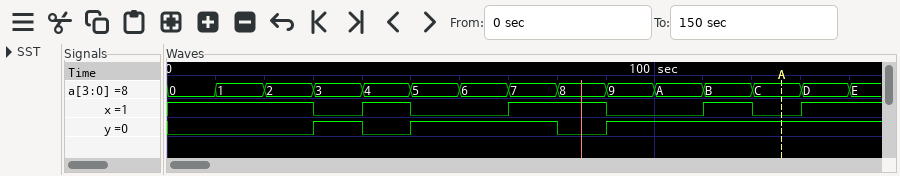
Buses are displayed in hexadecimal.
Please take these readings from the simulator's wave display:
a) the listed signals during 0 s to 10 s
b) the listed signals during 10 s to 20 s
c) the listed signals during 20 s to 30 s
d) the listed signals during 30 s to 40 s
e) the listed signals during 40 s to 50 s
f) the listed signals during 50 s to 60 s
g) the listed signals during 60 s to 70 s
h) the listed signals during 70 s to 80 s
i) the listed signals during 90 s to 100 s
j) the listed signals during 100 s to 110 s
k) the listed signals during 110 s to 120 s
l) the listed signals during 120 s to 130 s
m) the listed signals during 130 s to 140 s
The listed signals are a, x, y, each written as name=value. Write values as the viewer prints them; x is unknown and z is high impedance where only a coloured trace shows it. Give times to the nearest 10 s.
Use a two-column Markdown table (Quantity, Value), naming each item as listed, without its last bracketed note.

| Quantity | Value |
|---|---|
| the listed signals during 0 s to 10 s | a=0, x=1, y=0 |
| the listed signals during 10 s to 20 s | a=1, x=1, y=0 |
| the listed signals during 20 s to 30 s | a=2, x=1, y=0 |
| the listed signals during 30 s to 40 s | a=3, x=0, y=1 |
| the listed signals during 40 s to 50 s | a=4, x=1, y=0 |
| the listed signals during 50 s to 60 s | a=5, x=0, y=1 |
| the listed signals during 60 s to 70 s | a=6, x=0, y=1 |
| the listed signals during 70 s to 80 s | a=7, x=1, y=1 |
| the listed signals during 90 s to 100 s | a=9, x=0, y=1 |
| the listed signals during 100 s to 110 s | a=A, x=0, y=1 |
| the listed signals during 110 s to 120 s | a=B, x=1, y=1 |
| the listed signals during 120 s to 130 s | a=C, x=0, y=1 |
| the listed signals during 130 s to 140 s | a=D, x=1, y=1 |
